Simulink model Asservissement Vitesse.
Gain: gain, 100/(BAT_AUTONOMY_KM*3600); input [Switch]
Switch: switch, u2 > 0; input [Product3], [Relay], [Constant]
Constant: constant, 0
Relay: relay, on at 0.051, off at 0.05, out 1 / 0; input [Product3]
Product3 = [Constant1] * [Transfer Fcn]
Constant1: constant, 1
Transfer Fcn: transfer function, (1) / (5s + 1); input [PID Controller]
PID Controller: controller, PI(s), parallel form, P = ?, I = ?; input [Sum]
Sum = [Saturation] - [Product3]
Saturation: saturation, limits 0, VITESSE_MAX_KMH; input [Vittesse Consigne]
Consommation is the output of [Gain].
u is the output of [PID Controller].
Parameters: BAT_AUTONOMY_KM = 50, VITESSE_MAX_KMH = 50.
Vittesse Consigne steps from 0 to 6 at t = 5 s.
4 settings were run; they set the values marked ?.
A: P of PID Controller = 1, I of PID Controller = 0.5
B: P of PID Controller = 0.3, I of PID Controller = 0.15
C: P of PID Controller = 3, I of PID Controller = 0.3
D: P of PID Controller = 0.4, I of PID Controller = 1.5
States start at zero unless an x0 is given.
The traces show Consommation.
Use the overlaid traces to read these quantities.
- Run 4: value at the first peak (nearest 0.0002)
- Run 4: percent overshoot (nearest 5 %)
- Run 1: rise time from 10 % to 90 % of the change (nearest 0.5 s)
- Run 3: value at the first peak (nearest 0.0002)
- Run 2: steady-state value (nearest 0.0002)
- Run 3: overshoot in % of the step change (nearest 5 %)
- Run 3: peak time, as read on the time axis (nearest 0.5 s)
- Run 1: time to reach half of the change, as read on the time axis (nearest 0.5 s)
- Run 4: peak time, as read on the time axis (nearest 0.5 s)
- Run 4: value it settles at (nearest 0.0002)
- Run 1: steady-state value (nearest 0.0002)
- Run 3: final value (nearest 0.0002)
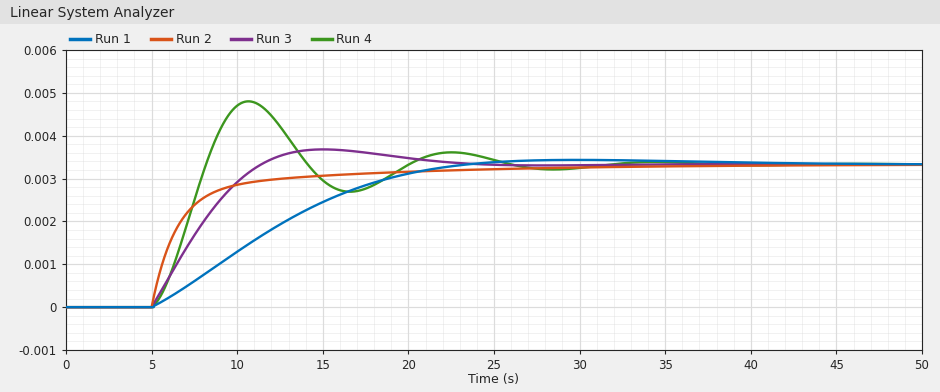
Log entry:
0.0048
45 %
12.5 s
0.0036
0.0034
10 %
15.0 s
11.5 s
10.5 s
0.0034
0.0034
0.0034
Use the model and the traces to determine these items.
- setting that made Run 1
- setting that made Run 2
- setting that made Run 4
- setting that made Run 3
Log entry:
B
C
D
A
